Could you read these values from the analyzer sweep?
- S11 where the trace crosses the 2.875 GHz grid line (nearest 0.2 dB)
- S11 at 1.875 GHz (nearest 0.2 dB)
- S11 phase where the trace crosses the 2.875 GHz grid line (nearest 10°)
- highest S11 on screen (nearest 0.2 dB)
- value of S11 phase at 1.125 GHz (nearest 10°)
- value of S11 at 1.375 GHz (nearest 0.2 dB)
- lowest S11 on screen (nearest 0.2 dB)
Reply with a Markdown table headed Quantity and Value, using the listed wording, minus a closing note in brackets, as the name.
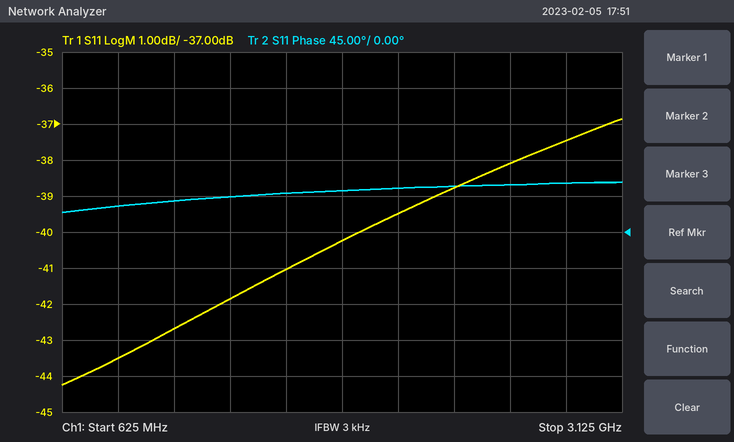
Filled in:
| Quantity | Value |
|---|---|
| S11 where the trace crosses the 2.875 GHz grid line | -37.4 dB |
| S11 at 1.875 GHz | -40.2 dB |
| S11 phase where the trace crosses the 2.875 GHz grid line | 60° |
| highest S11 on screen | -36.8 dB |
| value of S11 phase at 1.125 GHz | 40° |
| value of S11 at 1.375 GHz | -41.8 dB |
| lowest S11 on screen | -44.2 dB |
